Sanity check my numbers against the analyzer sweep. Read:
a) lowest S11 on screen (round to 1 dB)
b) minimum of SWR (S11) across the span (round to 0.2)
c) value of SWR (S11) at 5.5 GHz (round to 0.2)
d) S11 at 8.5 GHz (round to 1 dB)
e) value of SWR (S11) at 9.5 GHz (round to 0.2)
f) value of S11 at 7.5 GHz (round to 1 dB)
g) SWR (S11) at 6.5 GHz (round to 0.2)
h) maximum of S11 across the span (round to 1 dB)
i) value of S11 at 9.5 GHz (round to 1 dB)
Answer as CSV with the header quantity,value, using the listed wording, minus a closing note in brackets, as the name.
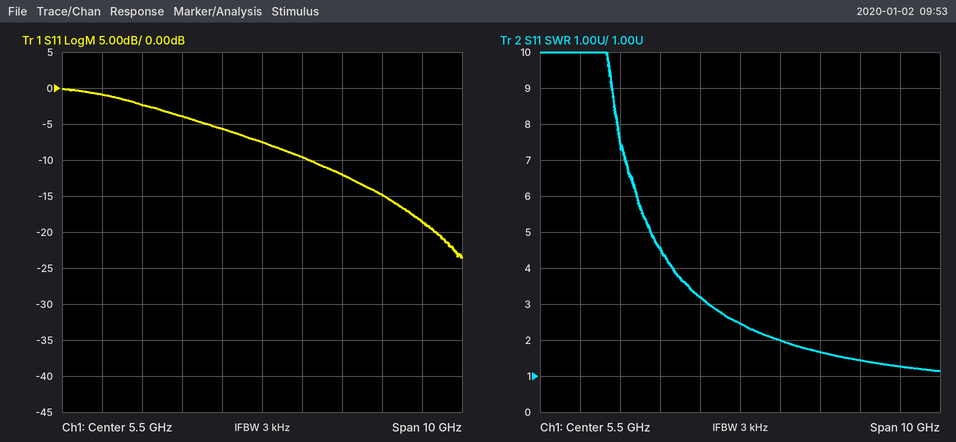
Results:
quantity,value
lowest S11 on screen,-24 dB
minimum of SWR (S11) across the span,1.2
value of SWR (S11) at 5.5 GHz,2.4
S11 at 8.5 GHz,-15 dB
value of SWR (S11) at 9.5 GHz,1.2
value of S11 at 7.5 GHz,-12 dB
SWR (S11) at 6.5 GHz,2.0
maximum of S11 across the span,0 dB
value of S11 at 9.5 GHz,-19 dB
